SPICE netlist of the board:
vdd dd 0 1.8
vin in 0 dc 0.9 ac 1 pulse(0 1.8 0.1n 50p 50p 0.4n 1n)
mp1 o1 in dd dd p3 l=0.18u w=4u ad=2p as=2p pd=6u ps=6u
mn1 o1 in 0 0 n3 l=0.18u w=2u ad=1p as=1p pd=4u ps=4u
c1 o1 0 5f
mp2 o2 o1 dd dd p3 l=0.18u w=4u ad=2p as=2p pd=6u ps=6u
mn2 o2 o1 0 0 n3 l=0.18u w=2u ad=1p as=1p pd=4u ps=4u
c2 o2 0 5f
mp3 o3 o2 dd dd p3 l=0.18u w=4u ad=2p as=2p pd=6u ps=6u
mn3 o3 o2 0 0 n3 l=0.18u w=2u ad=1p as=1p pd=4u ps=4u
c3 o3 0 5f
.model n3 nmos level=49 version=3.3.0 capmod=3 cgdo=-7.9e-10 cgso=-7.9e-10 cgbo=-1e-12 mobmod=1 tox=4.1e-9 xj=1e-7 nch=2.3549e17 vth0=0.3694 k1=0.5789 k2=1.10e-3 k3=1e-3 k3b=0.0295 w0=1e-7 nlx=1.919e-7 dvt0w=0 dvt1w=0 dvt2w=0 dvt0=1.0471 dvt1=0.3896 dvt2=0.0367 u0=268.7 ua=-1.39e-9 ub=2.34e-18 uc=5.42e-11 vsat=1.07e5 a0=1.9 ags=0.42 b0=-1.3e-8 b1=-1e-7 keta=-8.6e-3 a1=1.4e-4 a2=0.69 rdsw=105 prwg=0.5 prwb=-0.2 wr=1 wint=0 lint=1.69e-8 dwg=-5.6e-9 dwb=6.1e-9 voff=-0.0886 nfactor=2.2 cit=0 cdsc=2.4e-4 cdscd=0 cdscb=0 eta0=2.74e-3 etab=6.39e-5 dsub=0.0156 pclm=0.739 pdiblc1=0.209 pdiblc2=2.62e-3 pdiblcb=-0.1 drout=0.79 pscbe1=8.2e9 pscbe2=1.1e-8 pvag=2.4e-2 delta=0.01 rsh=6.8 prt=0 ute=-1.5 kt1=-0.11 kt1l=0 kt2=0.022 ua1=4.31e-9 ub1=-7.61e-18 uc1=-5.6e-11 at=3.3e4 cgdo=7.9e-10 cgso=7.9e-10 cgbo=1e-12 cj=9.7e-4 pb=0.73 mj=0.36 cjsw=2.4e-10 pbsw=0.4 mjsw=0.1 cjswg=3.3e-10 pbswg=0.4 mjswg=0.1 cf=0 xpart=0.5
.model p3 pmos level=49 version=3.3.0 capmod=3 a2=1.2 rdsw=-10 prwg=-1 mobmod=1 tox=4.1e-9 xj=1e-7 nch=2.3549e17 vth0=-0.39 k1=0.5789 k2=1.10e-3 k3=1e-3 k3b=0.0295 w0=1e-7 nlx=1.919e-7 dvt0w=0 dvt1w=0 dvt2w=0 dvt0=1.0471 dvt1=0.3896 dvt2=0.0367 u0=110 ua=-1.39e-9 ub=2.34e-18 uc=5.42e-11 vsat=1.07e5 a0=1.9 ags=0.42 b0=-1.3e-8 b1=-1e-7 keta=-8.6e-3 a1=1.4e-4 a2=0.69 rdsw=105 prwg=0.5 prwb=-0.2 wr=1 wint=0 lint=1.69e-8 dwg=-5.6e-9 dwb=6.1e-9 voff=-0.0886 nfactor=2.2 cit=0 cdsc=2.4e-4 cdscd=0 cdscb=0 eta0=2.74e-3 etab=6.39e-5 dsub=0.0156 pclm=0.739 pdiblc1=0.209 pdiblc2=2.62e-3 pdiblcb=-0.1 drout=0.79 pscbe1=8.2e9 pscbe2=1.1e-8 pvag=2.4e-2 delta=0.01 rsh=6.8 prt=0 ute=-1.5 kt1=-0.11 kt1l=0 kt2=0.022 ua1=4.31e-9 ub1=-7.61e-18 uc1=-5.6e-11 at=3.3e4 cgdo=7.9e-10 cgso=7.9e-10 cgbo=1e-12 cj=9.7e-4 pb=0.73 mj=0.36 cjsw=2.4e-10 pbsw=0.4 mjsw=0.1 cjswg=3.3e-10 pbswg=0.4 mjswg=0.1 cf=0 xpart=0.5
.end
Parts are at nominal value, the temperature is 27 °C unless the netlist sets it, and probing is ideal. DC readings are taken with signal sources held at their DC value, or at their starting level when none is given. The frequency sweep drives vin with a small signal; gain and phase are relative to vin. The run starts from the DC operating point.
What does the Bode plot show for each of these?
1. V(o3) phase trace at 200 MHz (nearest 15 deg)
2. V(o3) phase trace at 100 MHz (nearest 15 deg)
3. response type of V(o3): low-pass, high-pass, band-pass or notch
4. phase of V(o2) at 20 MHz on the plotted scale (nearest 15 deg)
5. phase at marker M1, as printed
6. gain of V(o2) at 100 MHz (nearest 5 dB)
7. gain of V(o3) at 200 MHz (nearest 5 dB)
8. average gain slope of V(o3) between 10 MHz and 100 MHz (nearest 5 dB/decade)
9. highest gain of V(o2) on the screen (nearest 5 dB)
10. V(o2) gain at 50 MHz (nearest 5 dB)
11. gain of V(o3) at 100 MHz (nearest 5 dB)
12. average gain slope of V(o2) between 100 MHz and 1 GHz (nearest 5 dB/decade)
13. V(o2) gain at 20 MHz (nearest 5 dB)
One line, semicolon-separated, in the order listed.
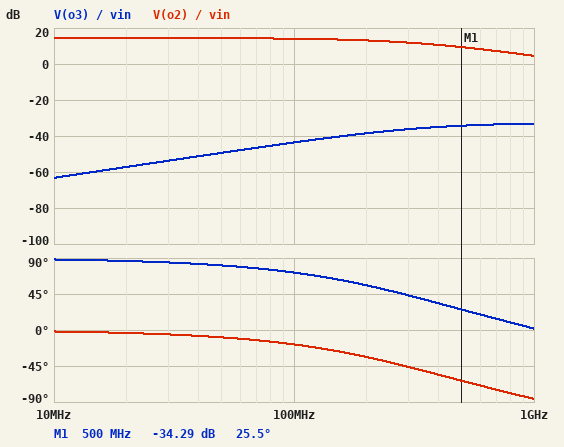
60 deg; 75 deg; high-pass; 0 deg; 25.5 deg; 15 dB; -40 dB; 20 dB/decade; 15 dB; 15 dB; -45 dB; -10 dB/decade; 15 dB
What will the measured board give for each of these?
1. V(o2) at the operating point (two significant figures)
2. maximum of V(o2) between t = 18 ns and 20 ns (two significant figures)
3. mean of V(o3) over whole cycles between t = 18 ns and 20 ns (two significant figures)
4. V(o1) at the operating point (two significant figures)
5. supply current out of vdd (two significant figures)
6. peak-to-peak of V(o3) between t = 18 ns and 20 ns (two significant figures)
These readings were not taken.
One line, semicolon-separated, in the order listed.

1.8 V; 1.9 V; 1.0 V; 610 mV; 200 µA; 2.0 V
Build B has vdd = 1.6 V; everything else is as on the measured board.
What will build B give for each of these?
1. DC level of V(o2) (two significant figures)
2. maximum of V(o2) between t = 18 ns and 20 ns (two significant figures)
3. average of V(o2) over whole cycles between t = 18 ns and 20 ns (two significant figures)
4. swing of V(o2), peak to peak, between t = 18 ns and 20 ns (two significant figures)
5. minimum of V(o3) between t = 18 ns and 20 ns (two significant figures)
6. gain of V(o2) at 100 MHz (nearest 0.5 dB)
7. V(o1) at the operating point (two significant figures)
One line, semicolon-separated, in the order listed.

1.6 V; 1.7 V; 730 mV; 1.8 V; -86 mV; -59.0 dB; 39 mV
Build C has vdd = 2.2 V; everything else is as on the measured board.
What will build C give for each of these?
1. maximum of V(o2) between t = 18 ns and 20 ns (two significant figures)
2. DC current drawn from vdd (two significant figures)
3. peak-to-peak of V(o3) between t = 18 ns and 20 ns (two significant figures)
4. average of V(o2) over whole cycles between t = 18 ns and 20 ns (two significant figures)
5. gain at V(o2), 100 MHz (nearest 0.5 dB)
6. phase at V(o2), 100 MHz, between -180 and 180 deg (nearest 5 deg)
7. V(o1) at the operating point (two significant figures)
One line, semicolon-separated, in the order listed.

2.3 V; 220 µA; 2.4 V; 950 mV; -60.5 dB; -90 deg; 2.1 V
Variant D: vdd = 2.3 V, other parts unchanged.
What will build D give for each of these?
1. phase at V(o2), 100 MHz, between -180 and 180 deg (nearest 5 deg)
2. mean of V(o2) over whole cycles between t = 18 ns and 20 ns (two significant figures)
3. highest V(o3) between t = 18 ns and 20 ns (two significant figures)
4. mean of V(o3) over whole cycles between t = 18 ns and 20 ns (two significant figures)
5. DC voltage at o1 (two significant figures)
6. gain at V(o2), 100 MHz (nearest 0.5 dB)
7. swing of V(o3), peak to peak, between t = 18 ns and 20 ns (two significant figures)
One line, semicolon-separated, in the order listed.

-90 deg; 990 mV; 2.4 V; 1.3 V; 2.2 V; -62.5 dB; 2.5 V
